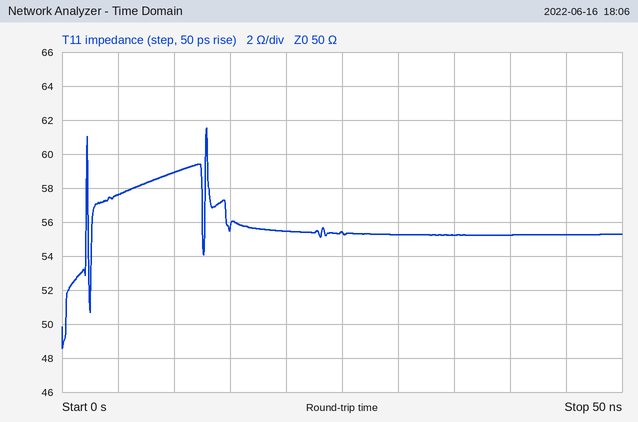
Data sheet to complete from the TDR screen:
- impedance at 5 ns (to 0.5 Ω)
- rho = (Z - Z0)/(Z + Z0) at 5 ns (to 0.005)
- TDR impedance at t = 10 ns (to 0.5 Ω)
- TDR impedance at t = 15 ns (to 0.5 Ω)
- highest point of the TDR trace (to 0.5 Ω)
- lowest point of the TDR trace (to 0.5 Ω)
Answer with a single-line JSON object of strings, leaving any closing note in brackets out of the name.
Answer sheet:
{"impedance at 5 ns": "57.5 Ω", "rho = (Z - Z0)/(Z + Z0) at 5 ns": "+0.070", "TDR impedance at t = 10 ns": "59.0 Ω", "TDR impedance at t = 15 ns": "55.5 Ω", "highest point of the TDR trace": "61.5 Ω", "lowest point of the TDR trace": "48.5 Ω"}
